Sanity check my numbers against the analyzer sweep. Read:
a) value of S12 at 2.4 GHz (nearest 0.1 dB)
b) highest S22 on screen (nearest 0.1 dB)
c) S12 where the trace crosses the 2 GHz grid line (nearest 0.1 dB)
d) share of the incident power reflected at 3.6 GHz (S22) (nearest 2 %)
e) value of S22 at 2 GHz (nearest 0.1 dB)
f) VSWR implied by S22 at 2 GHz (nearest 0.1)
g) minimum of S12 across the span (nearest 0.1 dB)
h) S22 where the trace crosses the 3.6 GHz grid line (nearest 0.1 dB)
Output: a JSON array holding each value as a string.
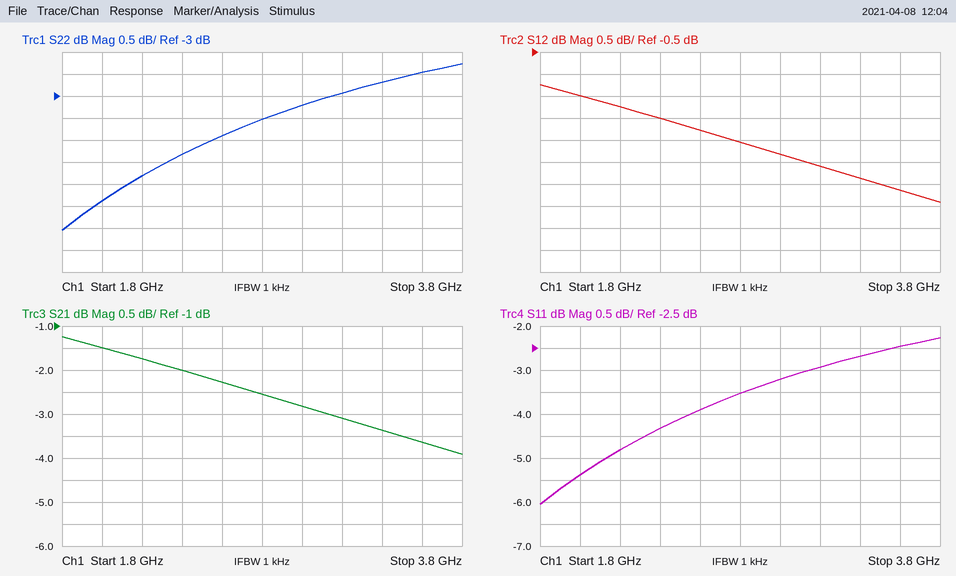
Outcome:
["-2.0 dB", "-2.3 dB", "-1.5 dB", "56 %", "-5.4 dB", "3.3", "-3.9 dB", "-2.5 dB"]
